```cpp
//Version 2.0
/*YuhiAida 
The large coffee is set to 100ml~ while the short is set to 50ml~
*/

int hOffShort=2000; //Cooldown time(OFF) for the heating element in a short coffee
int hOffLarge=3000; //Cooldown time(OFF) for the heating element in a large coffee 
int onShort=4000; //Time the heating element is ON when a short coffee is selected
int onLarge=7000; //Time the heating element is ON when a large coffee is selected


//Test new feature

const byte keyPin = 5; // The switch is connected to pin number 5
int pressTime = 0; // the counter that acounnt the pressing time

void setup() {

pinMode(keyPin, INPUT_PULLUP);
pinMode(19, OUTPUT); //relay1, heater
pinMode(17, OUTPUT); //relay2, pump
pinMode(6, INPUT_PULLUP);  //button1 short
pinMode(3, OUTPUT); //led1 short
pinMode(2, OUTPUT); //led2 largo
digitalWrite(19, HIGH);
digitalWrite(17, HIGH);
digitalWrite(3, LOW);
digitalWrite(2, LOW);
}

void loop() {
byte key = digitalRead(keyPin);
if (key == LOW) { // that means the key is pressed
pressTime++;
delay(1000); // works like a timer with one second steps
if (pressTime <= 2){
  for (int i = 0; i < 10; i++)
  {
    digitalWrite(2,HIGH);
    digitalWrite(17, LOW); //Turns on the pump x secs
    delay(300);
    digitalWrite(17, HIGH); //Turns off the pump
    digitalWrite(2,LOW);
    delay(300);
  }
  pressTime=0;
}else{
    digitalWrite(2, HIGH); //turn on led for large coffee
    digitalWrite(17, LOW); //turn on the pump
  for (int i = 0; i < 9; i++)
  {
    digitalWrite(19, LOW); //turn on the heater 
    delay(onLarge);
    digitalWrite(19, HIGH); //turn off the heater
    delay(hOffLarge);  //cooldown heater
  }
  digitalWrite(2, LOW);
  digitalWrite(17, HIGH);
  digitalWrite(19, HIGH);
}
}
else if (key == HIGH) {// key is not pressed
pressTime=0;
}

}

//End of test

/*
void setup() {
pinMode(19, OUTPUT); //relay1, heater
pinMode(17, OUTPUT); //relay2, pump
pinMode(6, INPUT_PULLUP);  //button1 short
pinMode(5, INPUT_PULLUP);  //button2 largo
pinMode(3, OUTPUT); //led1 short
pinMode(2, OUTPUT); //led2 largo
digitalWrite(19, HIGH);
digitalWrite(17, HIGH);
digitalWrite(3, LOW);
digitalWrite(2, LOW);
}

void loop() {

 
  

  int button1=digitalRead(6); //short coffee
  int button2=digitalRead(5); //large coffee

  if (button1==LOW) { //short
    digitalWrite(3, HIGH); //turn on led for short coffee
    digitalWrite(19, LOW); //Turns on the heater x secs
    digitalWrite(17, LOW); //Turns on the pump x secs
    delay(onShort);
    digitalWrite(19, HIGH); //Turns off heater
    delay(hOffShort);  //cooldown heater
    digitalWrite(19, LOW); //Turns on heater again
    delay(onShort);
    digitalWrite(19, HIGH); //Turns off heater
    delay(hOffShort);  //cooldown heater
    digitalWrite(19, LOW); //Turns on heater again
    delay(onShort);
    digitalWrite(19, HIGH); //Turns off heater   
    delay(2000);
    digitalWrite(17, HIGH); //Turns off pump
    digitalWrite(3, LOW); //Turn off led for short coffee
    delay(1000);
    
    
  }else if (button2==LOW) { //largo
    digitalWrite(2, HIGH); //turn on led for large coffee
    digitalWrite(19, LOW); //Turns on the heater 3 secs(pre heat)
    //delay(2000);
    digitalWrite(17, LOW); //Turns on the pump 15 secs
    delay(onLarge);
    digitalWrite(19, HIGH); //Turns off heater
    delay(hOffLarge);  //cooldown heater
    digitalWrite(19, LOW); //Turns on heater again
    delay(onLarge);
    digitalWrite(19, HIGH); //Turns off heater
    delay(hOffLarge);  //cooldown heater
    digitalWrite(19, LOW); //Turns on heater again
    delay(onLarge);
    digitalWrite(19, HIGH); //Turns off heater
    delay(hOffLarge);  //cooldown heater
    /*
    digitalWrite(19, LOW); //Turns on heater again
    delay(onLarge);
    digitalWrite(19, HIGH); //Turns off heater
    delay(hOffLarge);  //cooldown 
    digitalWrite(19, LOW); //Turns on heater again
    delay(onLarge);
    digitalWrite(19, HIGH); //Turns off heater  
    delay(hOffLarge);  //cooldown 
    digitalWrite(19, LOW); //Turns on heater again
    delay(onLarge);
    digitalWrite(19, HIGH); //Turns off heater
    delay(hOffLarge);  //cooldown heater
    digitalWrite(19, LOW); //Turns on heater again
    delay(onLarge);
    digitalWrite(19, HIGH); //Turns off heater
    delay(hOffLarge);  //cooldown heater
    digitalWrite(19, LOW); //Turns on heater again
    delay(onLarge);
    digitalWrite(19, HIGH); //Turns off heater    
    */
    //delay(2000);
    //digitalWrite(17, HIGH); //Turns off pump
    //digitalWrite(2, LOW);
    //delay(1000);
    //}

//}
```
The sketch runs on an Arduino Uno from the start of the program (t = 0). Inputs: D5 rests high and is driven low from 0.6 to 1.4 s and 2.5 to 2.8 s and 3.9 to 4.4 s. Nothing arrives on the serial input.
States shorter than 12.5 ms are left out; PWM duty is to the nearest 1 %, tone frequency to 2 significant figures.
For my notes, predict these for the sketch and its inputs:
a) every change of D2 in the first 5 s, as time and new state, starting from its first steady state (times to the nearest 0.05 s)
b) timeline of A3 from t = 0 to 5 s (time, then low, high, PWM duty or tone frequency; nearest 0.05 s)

0 s low; 1.6 s high; 1.9 s low; 2.2 s high; 2.5 s low; 2.8 s high; 3.1 s low; 3.4 s high; 3.7 s low; 4 s high; 4.3 s low; 4.6 s high; 4.9 s low
0 s high; 1.6 s low; 1.9 s high; 2.2 s low; 2.5 s high; 2.8 s low; 3.1 s high; 3.4 s low; 3.7 s high; 4 s low; 4.3 s high; 4.6 s low; 4.9 s high
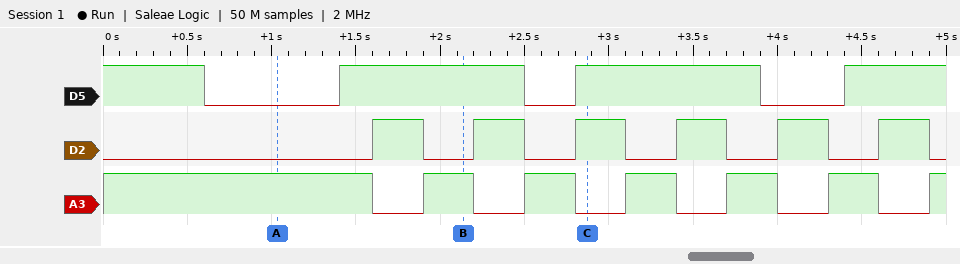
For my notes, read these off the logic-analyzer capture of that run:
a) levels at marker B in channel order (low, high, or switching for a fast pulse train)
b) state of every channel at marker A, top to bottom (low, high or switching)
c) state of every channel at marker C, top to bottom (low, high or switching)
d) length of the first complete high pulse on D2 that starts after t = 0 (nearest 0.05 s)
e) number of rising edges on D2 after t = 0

D5 high, D2 low, A3 high
D5 low, D2 low, A3 high
D5 high, D2 high, A3 low
0.30 s
6
